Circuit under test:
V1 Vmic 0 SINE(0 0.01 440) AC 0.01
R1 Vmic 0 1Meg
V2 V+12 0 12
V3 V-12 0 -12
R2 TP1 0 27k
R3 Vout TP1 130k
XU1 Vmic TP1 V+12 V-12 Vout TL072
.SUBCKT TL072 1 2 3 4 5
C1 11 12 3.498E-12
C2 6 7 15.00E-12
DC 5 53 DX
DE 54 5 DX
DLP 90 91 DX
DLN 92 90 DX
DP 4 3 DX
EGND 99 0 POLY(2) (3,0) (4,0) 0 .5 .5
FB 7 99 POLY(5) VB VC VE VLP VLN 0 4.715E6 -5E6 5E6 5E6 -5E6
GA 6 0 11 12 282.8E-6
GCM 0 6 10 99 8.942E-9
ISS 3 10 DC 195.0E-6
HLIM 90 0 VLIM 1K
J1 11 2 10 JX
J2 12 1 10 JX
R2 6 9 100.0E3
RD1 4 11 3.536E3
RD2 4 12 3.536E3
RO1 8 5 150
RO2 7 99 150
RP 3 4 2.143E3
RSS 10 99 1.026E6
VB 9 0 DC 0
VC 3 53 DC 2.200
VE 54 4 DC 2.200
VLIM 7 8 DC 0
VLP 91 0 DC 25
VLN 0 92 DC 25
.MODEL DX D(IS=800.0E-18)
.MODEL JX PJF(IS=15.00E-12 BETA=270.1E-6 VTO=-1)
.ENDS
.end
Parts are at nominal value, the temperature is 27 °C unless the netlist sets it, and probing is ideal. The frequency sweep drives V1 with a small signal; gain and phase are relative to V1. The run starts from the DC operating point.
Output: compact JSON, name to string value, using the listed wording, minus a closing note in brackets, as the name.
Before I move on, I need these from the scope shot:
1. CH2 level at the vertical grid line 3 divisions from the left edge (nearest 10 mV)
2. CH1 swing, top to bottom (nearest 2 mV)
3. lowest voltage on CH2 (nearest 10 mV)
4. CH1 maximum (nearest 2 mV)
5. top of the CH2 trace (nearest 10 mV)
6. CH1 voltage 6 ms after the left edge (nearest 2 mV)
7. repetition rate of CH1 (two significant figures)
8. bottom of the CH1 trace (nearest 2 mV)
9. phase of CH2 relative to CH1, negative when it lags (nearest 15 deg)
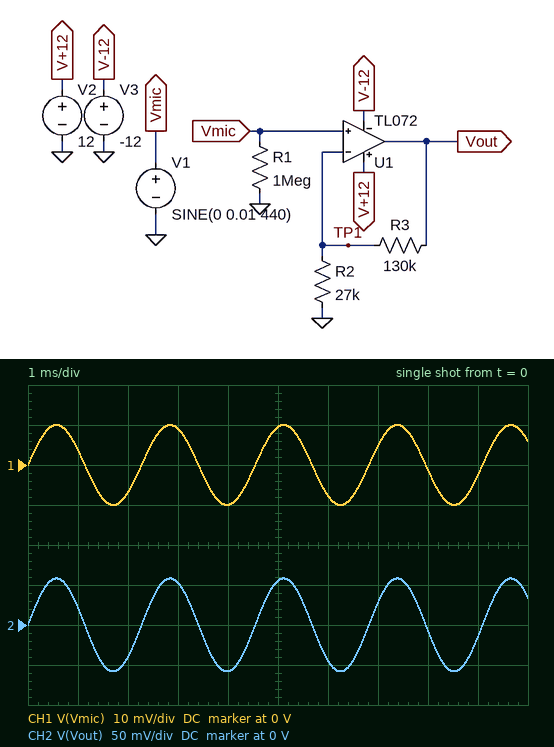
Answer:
{"CH2 level at the vertical grid line 3 divisions from the left edge": "50 mV", "CH1 swing, top to bottom": "20 mV", "lowest voltage on CH2": "-60 mV", "CH1 maximum": "10 mV", "top of the CH2 trace": "60 mV", "CH1 voltage 6 ms after the left edge": "-8 mV", "repetition rate of CH1": "440 Hz", "bottom of the CH1 trace": "-10 mV", "phase of CH2 relative to CH1, negative when it lags": "0 deg"}
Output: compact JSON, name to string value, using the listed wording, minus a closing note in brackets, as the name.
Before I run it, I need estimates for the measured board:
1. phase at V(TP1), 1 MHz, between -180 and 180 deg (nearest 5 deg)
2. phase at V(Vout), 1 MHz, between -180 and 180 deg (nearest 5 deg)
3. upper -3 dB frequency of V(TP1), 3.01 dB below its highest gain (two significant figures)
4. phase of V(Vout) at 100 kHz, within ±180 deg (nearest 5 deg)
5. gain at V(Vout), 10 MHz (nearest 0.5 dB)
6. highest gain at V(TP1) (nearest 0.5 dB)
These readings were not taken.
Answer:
{"phase at V(TP1), 1 MHz, between -180 and 180 deg": "-65 deg", "phase at V(Vout), 1 MHz, between -180 and 180 deg": "-65 deg", "upper -3 dB frequency of V(TP1), 3.01 dB below its highest gain": "650 kHz", "phase of V(Vout) at 100 kHz, within ±180 deg": "-10 deg", "gain at V(Vout), 10 MHz": "-14.5 dB", "highest gain at V(TP1)": "0 dB"}
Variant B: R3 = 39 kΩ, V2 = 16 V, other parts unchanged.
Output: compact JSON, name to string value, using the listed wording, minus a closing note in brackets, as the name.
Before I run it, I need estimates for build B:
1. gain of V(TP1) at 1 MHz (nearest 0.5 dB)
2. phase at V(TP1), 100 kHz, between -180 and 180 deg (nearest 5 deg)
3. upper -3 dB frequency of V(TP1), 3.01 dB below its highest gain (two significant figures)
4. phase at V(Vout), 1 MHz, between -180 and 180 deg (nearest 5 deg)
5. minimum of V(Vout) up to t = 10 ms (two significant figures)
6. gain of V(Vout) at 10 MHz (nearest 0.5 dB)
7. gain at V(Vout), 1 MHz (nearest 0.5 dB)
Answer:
{"gain of V(TP1) at 1 MHz": "-1.0 dB", "phase at V(TP1), 100 kHz, between -180 and 180 deg": "-5 deg", "upper -3 dB frequency of V(TP1), 3.01 dB below its highest gain": "1.8 MHz", "phase at V(Vout), 1 MHz, between -180 and 180 deg": "-40 deg", "minimum of V(Vout) up to t = 10 ms": "-24 mV", "gain of V(Vout) at 10 MHz": "-14.0 dB", "gain at V(Vout), 1 MHz": "6.5 dB"}
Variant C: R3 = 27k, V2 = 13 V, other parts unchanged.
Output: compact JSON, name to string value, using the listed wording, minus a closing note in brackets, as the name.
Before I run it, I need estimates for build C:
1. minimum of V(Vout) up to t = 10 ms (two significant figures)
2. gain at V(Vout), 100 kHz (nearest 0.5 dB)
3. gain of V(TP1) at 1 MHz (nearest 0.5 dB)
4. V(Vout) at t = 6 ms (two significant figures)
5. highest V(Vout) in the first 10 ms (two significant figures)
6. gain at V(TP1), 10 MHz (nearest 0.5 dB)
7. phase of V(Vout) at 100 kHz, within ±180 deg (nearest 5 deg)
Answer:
{"minimum of V(Vout) up to t = 10 ms": "-20 mV", "gain at V(Vout), 100 kHz": "6.0 dB", "gain of V(TP1) at 1 MHz": "-0.5 dB", "V(Vout) at t = 6 ms": "-15 mV", "highest V(Vout) in the first 10 ms": "20 mV", "gain at V(TP1), 10 MHz": "-20.0 dB", "phase of V(Vout) at 100 kHz, within ±180 deg": "-5 deg"}
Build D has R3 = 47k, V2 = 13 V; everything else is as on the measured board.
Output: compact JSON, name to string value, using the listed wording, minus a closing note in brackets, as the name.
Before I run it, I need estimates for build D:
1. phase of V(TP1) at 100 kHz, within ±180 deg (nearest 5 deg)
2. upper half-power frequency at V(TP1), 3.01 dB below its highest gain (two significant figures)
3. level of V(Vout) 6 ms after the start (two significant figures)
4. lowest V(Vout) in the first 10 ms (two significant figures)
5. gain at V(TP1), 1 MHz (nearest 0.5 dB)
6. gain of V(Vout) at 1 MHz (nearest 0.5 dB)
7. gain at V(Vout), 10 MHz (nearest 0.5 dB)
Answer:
{"phase of V(TP1) at 100 kHz, within ±180 deg": "-5 deg", "upper half-power frequency at V(TP1), 3.01 dB below its highest gain": "1.5 MHz", "level of V(Vout) 6 ms after the start": "-21 mV", "lowest V(Vout) in the first 10 ms": "-27 mV", "gain at V(TP1), 1 MHz": "-1.5 dB", "gain of V(Vout) at 1 MHz": "7.5 dB", "gain at V(Vout), 10 MHz": "-14.0 dB"}
